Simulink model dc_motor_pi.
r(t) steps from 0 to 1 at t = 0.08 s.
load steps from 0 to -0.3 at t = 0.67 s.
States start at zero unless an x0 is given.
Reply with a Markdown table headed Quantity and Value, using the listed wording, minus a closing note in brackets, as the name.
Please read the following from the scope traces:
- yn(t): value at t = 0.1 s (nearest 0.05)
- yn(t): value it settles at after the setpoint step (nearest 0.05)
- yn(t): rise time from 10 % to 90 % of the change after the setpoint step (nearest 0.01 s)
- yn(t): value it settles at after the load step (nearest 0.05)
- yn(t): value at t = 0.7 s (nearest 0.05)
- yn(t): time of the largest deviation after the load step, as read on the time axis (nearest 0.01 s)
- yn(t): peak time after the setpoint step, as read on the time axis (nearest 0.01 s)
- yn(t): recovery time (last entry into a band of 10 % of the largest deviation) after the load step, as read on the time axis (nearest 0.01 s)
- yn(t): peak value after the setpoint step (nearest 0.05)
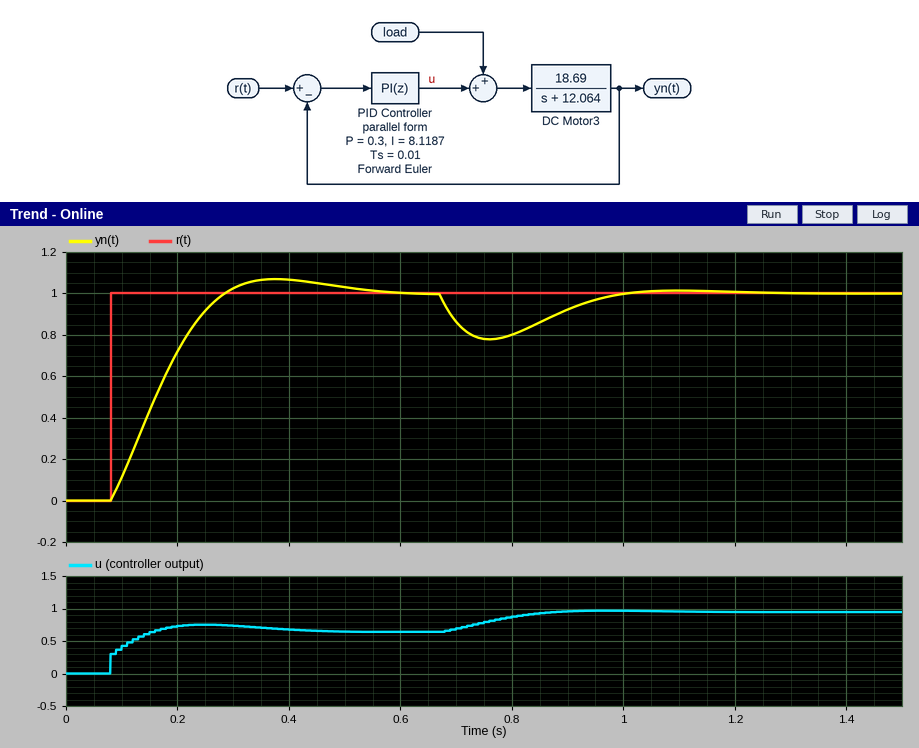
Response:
| Quantity | Value |
|---|---|
| yn(t): value at t = 0.1 s | 0.10 |
| yn(t): value it settles at after the setpoint step | 1.00 |
| yn(t): rise time from 10 % to 90 % of the change after the setpoint step | 0.15 s |
| yn(t): value it settles at after the load step | 1.00 |
| yn(t): value at t = 0.7 s | 0.85 |
| yn(t): time of the largest deviation after the load step, as read on the time axis | 0.76 s |
| yn(t): peak time after the setpoint step, as read on the time axis | 0.38 s |
| yn(t): recovery time (last entry into a band of 10 % of the largest deviation) after the load step, as read on the time axis | 0.96 s |
| yn(t): peak value after the setpoint step | 1.05 |
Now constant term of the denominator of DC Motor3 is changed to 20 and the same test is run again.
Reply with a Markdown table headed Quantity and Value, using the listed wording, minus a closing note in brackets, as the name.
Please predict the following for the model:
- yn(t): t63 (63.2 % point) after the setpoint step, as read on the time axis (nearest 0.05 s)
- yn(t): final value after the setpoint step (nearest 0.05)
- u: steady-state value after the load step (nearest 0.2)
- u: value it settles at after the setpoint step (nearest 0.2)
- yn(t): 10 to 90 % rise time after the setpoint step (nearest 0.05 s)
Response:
| Quantity | Value |
|---|---|
| yn(t): t63 (63.2 % point) after the setpoint step, as read on the time axis | 0.20 s |
| yn(t): final value after the setpoint step | 1.00 |
| u: steady-state value after the load step | 1.4 |
| u: value it settles at after the setpoint step | 1.0 |
| yn(t): 10 to 90 % rise time after the setpoint step | 0.25 s |
